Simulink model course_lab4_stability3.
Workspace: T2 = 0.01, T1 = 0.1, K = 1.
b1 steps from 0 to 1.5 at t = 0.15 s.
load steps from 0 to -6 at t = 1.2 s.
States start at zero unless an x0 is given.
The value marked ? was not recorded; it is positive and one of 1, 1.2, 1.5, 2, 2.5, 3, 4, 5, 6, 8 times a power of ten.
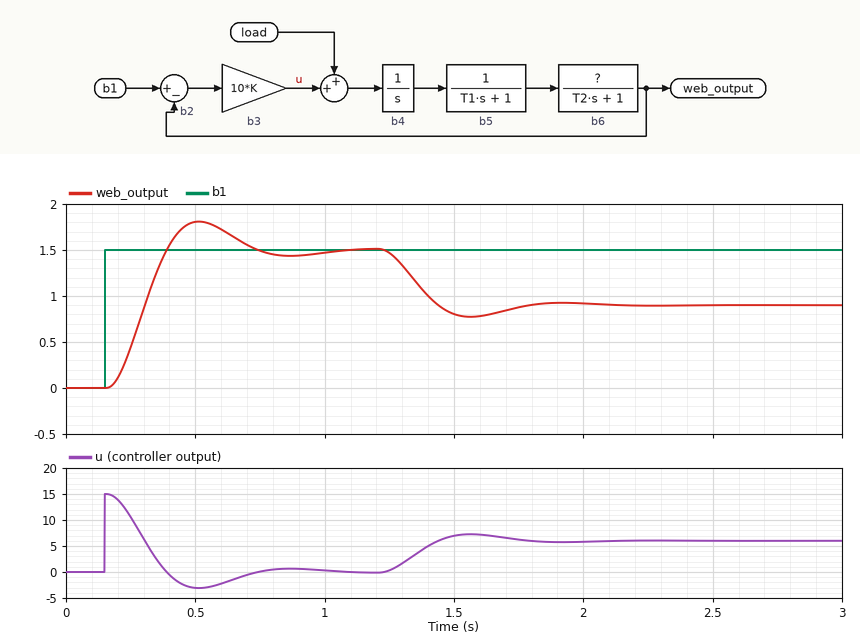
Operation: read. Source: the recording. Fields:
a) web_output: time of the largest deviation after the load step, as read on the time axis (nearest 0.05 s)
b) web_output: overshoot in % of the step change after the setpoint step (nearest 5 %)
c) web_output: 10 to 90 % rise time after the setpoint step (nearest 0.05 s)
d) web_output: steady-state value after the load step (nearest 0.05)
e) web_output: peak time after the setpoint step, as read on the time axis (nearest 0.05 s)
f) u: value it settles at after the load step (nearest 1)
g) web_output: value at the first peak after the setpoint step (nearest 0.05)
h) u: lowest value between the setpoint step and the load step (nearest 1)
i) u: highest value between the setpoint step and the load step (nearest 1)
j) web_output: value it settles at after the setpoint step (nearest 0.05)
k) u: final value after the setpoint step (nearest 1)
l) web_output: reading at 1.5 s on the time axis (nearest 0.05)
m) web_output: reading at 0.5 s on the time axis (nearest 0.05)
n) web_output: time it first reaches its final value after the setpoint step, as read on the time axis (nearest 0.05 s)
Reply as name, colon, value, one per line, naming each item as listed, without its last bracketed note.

web_output: time of the largest deviation after the load step, as read on the time axis: 1.55 s
web_output: overshoot in % of the step change after the setpoint step: 20 %
web_output: 10 to 90 % rise time after the setpoint step: 0.15 s
web_output: steady-state value after the load step: 0.90
web_output: peak time after the setpoint step, as read on the time axis: 0.50 s
u: value it settles at after the load step: 6
web_output: value at the first peak after the setpoint step: 1.80
u: lowest value between the setpoint step and the load step: -3
u: highest value between the setpoint step and the load step: 15
web_output: value it settles at after the setpoint step: 1.50
u: final value after the setpoint step: 0
web_output: reading at 1.5 s on the time axis: 0.80
web_output: reading at 0.5 s on the time axis: 1.80
web_output: time it first reaches its final value after the setpoint step, as read on the time axis: 0.40 s
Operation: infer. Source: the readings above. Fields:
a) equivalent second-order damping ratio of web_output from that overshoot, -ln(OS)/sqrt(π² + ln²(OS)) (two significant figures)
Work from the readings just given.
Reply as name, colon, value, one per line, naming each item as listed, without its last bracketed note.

equivalent second-order damping ratio of web_output from that overshoot, -ln(OS)/sqrt(π² + ln²(OS)): 0.46
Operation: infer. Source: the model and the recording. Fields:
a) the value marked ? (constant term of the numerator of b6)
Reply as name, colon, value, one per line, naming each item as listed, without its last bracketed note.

the value marked ?: 1
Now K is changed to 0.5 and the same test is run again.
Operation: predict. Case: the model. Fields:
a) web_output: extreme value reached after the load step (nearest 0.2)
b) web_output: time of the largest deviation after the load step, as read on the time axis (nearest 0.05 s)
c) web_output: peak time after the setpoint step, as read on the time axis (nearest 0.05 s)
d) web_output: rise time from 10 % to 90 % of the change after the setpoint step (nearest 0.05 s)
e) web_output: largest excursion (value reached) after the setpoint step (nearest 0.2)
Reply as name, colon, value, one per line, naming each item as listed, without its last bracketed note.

web_output: extreme value reached after the load step: 0.2
web_output: time of the largest deviation after the load step, as read on the time axis: 1.80 s
web_output: peak time after the setpoint step, as read on the time axis: 0.75 s
web_output: rise time from 10 % to 90 % of the change after the setpoint step: 0.30 s
web_output: largest excursion (value reached) after the setpoint step: 1.6
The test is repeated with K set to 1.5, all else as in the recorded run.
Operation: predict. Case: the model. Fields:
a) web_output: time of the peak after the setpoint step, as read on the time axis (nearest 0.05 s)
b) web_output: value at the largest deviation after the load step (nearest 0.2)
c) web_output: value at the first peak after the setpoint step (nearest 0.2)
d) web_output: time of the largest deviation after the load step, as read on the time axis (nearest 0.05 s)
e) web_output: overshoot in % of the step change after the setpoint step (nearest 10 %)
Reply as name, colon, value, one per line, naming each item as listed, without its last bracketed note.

web_output: time of the peak after the setpoint step, as read on the time axis: 0.45 s
web_output: value at the largest deviation after the load step: 1.0
web_output: value at the first peak after the setpoint step: 2.0
web_output: time of the largest deviation after the load step, as read on the time axis: 1.50 s
web_output: overshoot in % of the step change after the setpoint step: 30 %
